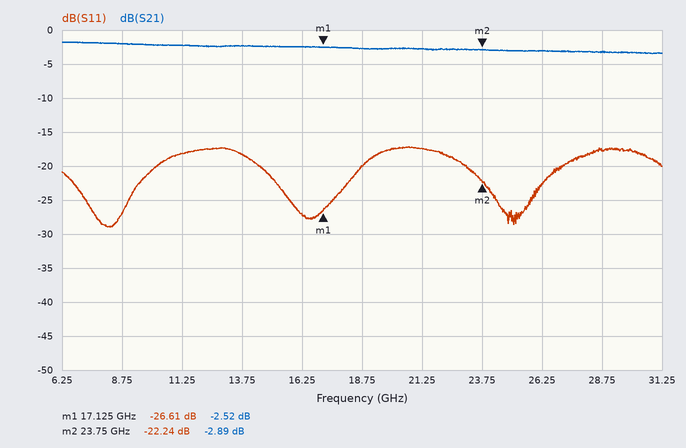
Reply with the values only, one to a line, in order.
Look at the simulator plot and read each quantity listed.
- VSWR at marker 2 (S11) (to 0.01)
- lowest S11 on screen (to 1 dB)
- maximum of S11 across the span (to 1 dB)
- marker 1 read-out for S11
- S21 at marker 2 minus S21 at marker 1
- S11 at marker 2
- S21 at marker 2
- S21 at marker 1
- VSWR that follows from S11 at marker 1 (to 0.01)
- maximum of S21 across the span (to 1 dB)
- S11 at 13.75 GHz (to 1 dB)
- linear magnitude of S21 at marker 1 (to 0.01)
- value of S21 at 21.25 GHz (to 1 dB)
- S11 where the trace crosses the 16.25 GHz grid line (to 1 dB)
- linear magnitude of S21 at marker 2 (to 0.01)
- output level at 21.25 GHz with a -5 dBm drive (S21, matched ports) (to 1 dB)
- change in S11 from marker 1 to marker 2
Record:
1.17
-29 dB
-17 dB
-26.61 dB
-0.37 dB
-22.24 dB
-2.89 dB
-2.52 dB
1.10
-2 dB
-18 dB
0.75
-3 dB
-27 dB
0.72
-8 dBm
4.37 dB
